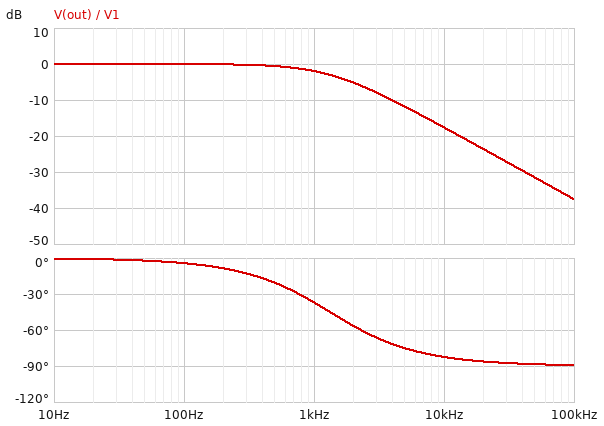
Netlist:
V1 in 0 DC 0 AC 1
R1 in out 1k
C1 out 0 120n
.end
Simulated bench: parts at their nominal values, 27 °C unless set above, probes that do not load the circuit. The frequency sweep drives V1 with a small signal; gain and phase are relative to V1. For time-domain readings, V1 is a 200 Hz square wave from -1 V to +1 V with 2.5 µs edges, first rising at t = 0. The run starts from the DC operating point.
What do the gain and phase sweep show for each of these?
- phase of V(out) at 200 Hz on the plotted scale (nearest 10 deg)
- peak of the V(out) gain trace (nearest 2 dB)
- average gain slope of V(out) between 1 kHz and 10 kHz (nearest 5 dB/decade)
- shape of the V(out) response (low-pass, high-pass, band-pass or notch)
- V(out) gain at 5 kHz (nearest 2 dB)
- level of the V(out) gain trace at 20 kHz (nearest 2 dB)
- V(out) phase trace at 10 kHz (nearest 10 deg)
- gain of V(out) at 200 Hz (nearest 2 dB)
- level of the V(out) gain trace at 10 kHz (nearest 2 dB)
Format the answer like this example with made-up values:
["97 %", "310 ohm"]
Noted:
["-10 deg", "0 dB", "-15 dB/decade", "low-pass", "-12 dB", "-24 dB", "-80 deg", "0 dB", "-18 dB"]
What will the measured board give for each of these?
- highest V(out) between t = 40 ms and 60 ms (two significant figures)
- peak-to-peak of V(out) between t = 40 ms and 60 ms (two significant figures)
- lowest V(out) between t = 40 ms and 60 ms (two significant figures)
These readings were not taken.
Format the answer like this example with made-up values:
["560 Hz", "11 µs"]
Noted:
["1.0 V", "2.0 V", "-1.0 V"]
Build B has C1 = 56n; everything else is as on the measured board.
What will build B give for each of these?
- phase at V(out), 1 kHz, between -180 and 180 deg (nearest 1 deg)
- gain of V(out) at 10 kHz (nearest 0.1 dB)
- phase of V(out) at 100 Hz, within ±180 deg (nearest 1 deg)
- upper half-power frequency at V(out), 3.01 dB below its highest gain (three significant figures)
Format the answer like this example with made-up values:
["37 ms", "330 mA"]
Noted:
["-19 deg", "-11.3 dB", "-2 deg", "2.84 kHz"]
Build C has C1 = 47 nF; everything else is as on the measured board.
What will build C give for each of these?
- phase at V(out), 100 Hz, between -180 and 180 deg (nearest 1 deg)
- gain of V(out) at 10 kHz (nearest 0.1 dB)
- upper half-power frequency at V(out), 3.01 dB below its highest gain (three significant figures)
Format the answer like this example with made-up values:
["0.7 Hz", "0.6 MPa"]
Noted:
["-2 deg", "-9.9 dB", "3.39 kHz"]
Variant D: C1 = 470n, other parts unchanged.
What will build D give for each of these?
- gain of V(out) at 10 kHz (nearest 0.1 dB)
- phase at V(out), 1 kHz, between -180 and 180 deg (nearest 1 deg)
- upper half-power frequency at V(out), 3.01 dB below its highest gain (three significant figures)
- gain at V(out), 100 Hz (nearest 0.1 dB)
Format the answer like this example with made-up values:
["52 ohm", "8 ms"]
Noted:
["-29.4 dB", "-71 deg", "339 Hz", "-0.4 dB"]
